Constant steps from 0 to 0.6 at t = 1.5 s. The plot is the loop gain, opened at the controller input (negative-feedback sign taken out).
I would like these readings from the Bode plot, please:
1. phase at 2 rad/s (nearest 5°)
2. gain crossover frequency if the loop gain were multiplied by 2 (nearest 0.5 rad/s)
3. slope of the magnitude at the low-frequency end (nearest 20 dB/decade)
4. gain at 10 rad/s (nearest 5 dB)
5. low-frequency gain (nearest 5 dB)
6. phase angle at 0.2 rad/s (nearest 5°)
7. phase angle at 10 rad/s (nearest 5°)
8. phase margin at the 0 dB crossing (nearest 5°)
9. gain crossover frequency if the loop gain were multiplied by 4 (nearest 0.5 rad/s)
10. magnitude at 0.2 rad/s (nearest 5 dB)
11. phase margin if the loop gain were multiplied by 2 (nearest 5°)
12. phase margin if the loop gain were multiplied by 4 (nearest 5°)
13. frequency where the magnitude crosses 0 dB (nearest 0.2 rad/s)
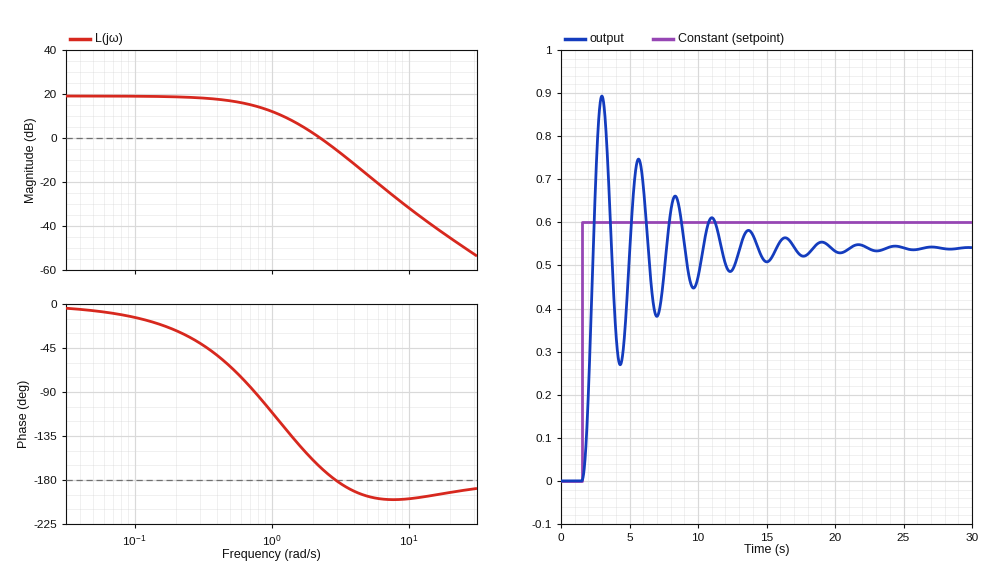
-160°
3.0 rad/s
0 dB/decade
-30 dB
20 dB
-25°
-200°
15°
4.0 rad/s
20 dB
0°
-10°
2.2 rad/s
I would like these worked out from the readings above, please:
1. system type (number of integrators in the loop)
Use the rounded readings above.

0
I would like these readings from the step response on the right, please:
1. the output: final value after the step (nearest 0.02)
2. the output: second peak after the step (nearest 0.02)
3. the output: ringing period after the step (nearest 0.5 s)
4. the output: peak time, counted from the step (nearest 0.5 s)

0.54
0.74
2.5 s
1.5 s
